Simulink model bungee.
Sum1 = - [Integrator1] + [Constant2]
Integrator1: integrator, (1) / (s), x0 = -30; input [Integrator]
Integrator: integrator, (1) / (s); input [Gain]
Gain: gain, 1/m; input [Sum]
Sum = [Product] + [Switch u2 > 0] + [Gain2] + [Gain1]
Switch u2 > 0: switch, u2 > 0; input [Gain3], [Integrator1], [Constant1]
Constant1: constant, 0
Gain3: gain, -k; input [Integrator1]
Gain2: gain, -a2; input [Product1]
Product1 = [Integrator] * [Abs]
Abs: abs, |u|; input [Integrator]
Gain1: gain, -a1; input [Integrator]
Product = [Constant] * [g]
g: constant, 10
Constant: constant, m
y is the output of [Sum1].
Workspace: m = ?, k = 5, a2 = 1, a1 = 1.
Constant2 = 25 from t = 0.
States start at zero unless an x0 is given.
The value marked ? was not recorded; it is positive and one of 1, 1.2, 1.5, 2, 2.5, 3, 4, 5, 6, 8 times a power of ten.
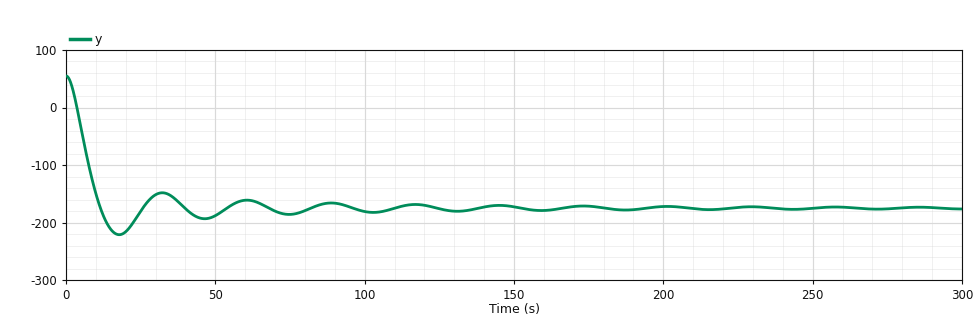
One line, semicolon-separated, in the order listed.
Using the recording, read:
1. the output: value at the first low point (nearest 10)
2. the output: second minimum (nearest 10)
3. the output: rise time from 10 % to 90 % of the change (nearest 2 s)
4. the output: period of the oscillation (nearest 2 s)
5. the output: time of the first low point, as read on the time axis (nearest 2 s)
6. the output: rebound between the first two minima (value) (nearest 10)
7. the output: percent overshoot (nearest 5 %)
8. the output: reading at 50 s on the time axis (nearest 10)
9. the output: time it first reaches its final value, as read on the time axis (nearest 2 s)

-220; -190; 8 s; 28 s; 18 s; -150; 20 %; -190; 12 s
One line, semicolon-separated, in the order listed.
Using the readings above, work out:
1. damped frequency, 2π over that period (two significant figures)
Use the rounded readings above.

0.22 rad/s
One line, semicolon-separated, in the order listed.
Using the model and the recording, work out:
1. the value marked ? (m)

100
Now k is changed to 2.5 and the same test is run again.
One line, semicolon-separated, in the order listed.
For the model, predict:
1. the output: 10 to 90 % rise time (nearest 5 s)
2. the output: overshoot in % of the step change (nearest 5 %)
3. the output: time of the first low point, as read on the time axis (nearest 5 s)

15 s; 10 %; 30 s
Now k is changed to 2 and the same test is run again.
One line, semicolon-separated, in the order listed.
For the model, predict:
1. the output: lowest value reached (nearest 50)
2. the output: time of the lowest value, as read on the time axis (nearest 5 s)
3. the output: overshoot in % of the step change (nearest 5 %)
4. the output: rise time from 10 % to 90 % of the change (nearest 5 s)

-500; 35 s; 10 %; 20 s
